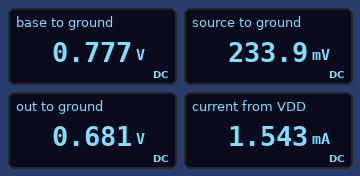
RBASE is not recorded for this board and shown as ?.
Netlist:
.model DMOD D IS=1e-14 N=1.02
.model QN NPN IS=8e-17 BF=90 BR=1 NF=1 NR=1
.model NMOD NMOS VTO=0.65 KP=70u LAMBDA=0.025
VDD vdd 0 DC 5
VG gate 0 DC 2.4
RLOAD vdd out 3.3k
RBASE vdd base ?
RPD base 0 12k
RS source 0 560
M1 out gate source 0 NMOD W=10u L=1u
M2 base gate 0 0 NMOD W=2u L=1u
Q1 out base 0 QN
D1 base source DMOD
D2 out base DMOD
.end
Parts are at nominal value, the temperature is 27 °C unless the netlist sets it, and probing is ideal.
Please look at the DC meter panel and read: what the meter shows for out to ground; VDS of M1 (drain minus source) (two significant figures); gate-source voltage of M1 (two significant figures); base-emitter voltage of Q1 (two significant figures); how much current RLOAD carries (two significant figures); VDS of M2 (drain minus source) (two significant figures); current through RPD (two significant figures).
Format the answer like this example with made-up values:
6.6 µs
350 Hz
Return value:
0.681 V
450 mV
2.2 V
780 mV
1.3 mA
780 mV
65 µA
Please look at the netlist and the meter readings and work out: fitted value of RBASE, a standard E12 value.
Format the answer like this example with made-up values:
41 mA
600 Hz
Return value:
18 kΩ
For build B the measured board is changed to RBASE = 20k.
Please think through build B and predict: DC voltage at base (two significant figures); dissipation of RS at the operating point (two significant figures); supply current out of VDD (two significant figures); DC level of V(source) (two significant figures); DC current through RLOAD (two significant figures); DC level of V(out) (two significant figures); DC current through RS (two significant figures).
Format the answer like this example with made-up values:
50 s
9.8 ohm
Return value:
760 mV
220 µW
1.3 mA
350 mV
1.1 mA
1.3 V
630 µA
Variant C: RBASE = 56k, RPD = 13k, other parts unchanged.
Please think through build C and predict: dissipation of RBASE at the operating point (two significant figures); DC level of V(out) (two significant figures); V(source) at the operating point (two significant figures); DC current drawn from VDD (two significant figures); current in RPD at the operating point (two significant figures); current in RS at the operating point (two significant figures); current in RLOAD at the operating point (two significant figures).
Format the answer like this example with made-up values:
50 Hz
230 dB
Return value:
320 µW
1.4 V
360 mV
1.2 mA
58 µA
640 µA
1.1 mA
